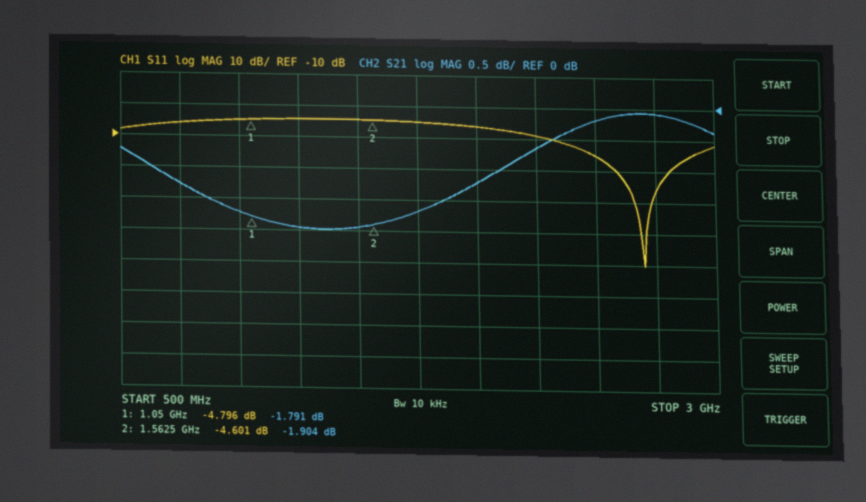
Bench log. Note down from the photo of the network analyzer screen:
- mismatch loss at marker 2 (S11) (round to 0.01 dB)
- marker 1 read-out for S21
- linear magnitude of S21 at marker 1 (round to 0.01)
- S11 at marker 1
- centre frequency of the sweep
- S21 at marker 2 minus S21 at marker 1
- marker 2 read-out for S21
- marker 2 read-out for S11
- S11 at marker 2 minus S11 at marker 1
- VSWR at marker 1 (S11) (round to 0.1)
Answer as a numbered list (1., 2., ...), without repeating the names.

1. 1.85 dB
2. -1.791 dB
3. 0.81
4. -4.796 dB
5. 1.75 GHz
6. -0.113 dB
7. -1.904 dB
8. -4.601 dB
9. 0.195 dB
10. 3.7
